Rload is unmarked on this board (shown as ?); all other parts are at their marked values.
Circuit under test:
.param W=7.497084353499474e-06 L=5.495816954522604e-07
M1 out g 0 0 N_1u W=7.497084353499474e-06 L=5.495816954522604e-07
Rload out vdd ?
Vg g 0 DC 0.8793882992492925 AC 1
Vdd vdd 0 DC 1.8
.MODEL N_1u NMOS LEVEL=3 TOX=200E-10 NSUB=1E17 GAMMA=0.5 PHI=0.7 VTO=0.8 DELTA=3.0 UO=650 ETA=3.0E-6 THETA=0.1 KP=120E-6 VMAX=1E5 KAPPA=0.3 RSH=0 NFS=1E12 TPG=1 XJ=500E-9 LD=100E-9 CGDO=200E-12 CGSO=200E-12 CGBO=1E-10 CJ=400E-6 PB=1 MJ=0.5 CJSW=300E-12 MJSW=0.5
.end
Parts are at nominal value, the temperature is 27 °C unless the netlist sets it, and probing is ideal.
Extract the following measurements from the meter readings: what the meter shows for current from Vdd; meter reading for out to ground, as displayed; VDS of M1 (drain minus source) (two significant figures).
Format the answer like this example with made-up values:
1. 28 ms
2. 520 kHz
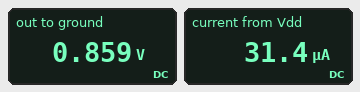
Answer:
1. 31.4 µA
2. 0.859 V
3. 860 mV
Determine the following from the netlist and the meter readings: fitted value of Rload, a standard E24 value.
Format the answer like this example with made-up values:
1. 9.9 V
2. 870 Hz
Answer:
1. 30 kΩ
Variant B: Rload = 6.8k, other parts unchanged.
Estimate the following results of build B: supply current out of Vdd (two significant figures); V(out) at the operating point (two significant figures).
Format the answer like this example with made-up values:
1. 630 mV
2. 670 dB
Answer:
1. 34 µA
2. 1.6 V
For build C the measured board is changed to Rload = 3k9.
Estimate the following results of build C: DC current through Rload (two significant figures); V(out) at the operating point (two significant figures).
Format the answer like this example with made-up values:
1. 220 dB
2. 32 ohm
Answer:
1. 34 µA
2. 1.7 V
